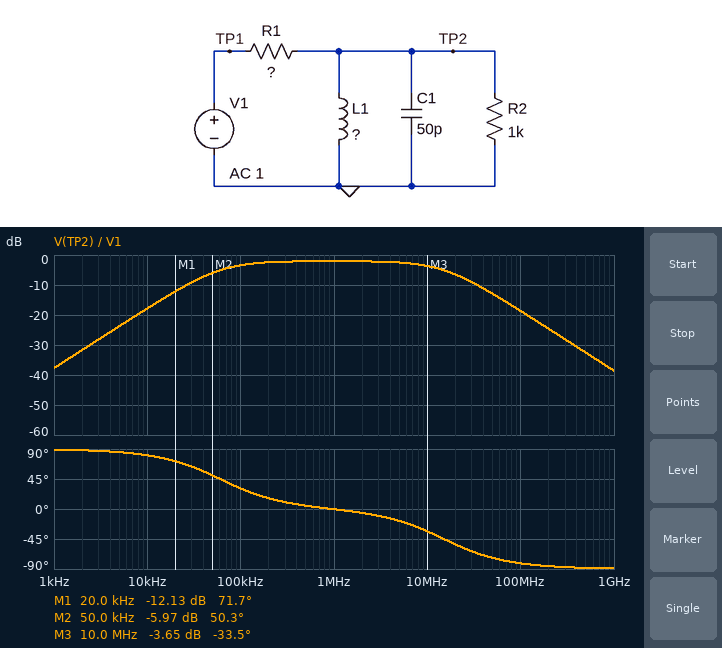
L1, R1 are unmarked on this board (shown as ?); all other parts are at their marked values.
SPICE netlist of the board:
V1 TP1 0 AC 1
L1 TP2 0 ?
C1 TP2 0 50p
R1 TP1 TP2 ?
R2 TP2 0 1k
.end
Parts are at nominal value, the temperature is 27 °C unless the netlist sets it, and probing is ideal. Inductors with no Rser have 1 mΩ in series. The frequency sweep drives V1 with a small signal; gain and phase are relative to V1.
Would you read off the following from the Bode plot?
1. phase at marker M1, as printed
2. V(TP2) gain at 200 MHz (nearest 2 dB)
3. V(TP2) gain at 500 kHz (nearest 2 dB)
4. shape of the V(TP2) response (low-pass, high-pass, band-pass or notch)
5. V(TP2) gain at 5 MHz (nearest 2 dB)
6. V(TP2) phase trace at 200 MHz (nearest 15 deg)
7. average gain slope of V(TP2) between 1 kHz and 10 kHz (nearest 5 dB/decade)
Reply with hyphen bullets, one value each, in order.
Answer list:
- 71.7 deg
- -24 dB
- -2 dB
- band-pass
- -2 dB
- -90 deg
- 20 dB/decade
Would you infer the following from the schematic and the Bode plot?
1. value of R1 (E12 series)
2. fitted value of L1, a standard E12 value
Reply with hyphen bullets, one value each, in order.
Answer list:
- 270 Ω
- 560 µH
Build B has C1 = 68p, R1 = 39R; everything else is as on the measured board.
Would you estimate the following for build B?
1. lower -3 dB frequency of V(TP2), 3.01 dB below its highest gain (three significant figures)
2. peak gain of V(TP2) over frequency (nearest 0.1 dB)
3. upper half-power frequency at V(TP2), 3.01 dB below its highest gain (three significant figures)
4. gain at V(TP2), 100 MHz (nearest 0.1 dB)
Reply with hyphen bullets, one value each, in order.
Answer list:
- 10.7 kHz
- -0.3 dB
- 62.4 MHz
- -5.9 dB
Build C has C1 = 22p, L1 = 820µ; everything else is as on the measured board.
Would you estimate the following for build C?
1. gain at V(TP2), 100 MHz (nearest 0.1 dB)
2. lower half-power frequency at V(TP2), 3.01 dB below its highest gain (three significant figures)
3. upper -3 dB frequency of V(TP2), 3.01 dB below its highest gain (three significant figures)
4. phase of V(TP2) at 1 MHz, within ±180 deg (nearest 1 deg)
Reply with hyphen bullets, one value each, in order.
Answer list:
- -11.9 dB
- 41.2 kHz
- 34.1 MHz
- 1 deg
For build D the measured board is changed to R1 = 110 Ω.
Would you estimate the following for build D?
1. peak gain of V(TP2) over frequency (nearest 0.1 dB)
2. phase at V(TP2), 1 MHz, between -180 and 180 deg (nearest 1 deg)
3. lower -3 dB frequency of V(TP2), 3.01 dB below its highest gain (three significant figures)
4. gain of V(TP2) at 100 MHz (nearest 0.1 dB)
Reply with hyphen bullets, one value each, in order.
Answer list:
- -0.9 dB
- 0 deg
- 28.1 kHz
- -11.2 dB
